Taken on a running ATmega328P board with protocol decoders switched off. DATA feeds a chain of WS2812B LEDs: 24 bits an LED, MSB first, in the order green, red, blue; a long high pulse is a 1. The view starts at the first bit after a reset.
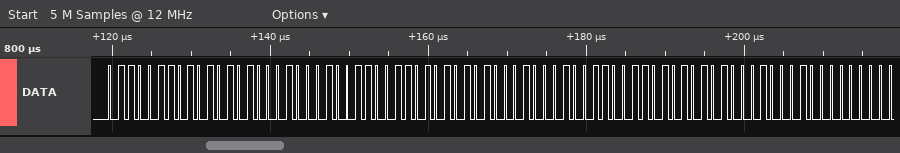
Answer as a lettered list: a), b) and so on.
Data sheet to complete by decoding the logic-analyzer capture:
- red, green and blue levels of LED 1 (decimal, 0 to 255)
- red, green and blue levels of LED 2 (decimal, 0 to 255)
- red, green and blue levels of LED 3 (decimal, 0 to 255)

a) 170, 102, 34
b) 170, 102, 34
c) 170, 102, 34
